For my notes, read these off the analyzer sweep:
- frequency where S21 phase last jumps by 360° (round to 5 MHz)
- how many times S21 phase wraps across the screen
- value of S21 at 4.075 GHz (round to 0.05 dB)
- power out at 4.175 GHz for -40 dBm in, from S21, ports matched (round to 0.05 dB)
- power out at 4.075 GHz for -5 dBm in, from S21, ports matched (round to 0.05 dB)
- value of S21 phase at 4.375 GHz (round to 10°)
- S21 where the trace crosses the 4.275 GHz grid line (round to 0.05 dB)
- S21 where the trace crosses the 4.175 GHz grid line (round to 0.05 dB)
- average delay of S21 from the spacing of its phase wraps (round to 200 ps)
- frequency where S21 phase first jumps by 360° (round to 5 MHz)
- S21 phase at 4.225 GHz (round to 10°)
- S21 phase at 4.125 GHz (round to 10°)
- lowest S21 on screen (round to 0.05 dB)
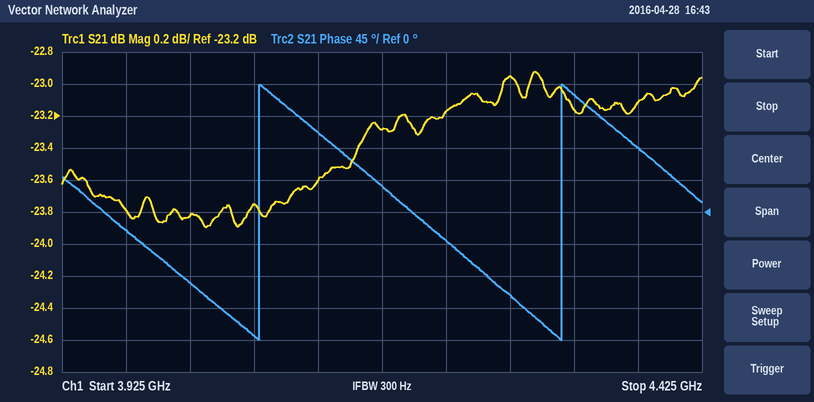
4.315 GHz
2
-23.75 dB
-63.30 dBm
-28.75 dBm
90°
-22.95 dB
-23.30 dB
4.2 ns
4.080 GHz
-40°
110°
-23.90 dB
